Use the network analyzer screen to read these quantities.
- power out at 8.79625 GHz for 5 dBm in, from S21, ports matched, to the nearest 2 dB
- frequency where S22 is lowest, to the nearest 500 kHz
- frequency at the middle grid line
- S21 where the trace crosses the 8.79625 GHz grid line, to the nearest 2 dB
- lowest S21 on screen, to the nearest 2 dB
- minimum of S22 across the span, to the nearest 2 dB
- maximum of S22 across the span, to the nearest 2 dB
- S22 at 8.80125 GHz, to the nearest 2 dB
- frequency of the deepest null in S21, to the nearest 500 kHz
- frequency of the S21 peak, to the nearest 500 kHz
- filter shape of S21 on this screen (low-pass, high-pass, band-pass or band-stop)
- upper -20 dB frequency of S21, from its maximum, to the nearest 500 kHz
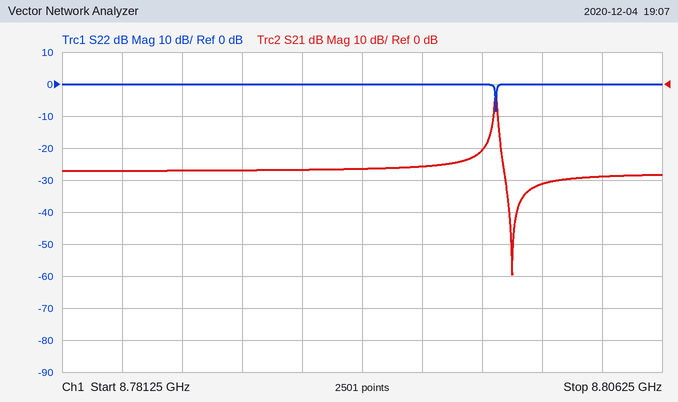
-20 dBm
8.7995 GHz
8.79375 GHz
-26 dB
-60 dB
-8 dB
0 dB
0 dB
8.8000 GHz
8.7995 GHz
band-pass
8.7995 GHz
